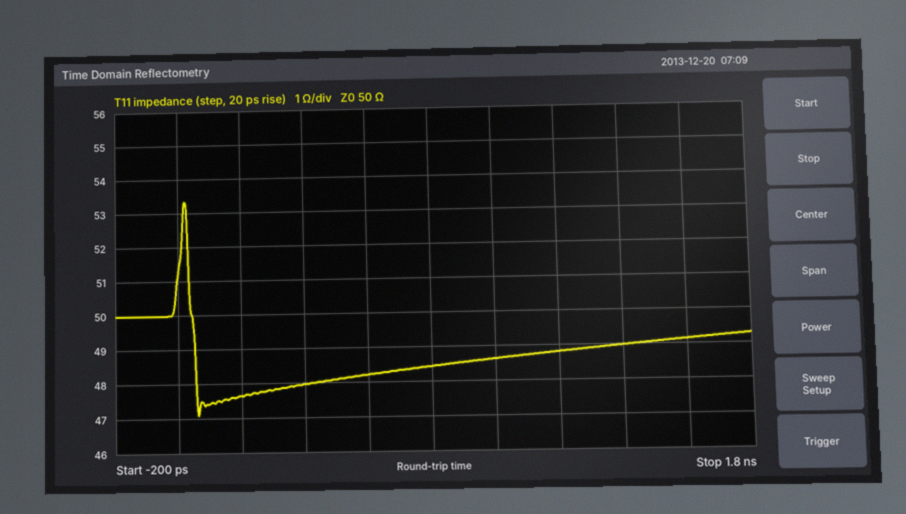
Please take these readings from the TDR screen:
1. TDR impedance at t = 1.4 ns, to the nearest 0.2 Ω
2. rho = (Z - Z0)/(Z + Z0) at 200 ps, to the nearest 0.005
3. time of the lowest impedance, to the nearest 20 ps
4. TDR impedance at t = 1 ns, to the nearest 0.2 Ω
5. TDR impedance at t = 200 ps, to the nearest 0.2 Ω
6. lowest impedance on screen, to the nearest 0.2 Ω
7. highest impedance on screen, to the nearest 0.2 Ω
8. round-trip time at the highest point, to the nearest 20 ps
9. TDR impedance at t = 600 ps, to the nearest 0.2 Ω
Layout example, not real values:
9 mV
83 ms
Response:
49.0 Ω
-0.025
60 ps
48.6 Ω
47.6 Ω
47.0 Ω
53.4 Ω
20 ps
48.2 Ω
